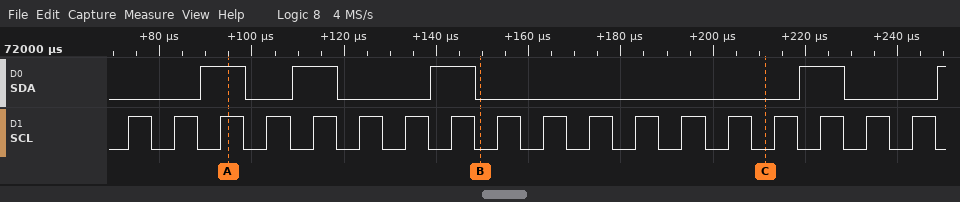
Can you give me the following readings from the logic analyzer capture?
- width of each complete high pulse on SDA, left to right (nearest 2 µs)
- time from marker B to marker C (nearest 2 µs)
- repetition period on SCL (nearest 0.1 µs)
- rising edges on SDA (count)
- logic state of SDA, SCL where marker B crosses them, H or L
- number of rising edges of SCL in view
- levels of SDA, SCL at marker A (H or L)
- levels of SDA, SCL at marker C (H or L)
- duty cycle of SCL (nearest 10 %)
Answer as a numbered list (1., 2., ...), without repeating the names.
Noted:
1. 10 µs, 10 µs, 10 µs, 10 µs
2. 62 µs
3. 10 µs
4. 5
5. SDA=L, SCL=L
6. 18
7. SDA=H, SCL=H
8. SDA=L, SCL=L
9. 50 %
